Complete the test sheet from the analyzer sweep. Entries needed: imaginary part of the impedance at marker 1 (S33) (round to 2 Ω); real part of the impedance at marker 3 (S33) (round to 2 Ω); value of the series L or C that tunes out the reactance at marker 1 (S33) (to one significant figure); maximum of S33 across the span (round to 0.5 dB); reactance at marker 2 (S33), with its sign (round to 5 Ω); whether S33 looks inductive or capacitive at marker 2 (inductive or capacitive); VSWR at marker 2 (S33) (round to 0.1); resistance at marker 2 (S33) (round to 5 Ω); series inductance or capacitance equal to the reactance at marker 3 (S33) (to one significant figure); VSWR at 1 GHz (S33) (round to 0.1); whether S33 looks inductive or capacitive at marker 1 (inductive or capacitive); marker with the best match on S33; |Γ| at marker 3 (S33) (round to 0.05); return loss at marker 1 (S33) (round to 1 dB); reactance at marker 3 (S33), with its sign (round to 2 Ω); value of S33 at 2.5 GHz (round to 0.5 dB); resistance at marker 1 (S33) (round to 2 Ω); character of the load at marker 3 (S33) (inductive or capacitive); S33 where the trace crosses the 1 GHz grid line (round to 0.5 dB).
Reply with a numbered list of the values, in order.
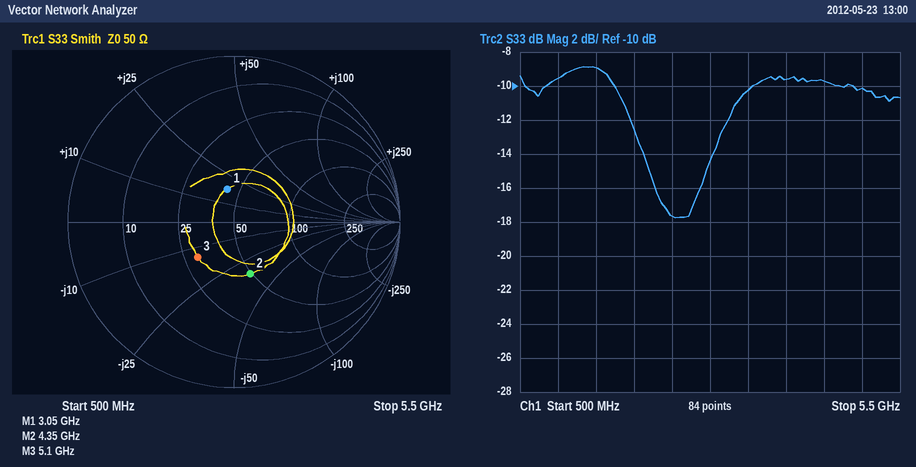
1. +18 Ω
2. 30 Ω
3. 3 pF
4. -9.0 dB
5. -35 Ω
6. capacitive
7. 2.0
8. 50 Ω
9. 2 pF
10. 2.0
11. inductive
12. marker 1
13. 0.30
14. 14 dB
15. -14 Ω
16. -17.5 dB
17. 42 Ω
18. capacitive
19. -9.5 dB
